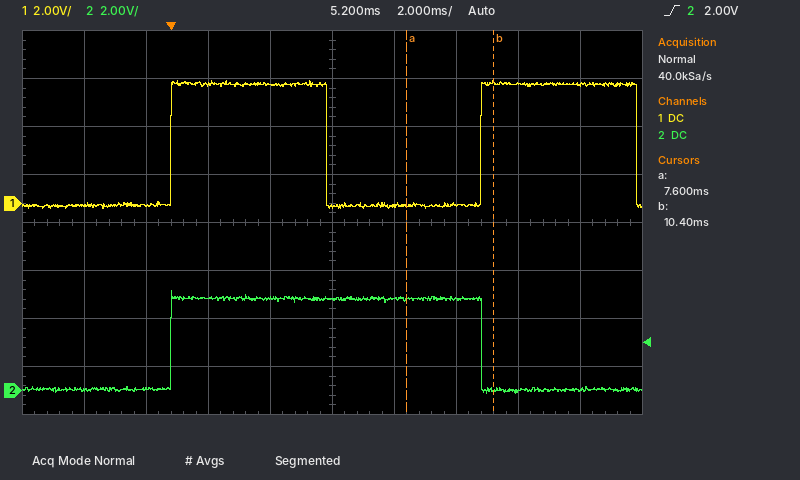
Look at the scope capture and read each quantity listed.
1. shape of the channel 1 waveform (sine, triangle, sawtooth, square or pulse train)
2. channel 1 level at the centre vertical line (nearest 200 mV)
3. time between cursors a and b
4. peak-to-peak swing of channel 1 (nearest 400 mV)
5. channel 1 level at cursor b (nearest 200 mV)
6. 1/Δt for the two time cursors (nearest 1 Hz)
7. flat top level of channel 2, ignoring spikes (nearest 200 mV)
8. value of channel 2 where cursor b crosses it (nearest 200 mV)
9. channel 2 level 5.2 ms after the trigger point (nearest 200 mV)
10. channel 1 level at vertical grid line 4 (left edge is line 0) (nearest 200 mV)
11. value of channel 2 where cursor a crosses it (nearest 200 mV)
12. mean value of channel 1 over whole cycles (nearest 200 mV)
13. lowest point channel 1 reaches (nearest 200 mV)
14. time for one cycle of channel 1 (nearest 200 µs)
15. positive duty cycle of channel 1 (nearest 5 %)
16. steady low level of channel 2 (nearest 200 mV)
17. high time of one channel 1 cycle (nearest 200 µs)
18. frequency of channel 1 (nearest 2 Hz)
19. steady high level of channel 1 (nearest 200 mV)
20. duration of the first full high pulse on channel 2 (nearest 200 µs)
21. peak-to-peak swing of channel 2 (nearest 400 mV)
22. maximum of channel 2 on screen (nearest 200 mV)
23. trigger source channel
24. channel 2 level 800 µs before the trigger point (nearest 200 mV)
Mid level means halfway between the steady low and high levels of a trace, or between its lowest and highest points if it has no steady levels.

square
-200 mV
2.8 ms
5.2 V
5.0 V
357 Hz
3.8 V
0.0 V
3.8 V
5.0 V
3.8 V
2.4 V
-200 mV
10.0 ms
50 %
0.0 V
5.0 ms
100 Hz
5.0 V
10.0 ms
4.4 V
4.2 V
channel 2
0.0 V
